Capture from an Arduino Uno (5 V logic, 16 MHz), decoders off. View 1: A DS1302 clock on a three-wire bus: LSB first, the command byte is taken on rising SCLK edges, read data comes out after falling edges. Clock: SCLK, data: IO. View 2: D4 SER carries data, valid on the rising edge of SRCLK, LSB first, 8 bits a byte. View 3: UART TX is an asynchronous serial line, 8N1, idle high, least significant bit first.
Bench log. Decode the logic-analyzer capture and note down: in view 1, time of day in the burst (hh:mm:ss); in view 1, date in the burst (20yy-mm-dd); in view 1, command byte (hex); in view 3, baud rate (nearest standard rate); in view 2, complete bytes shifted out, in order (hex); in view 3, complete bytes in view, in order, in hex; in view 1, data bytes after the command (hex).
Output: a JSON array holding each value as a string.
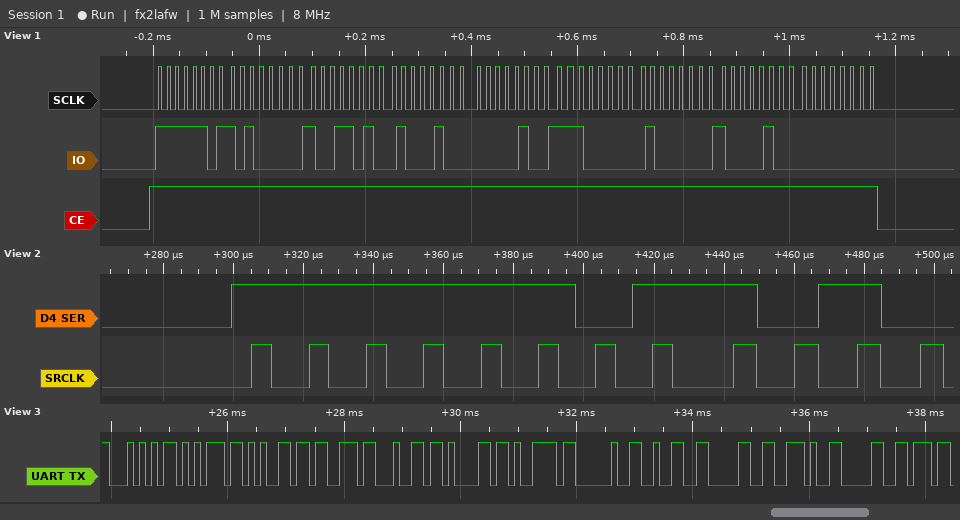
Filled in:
["22:59:05", "2021-07-20", "0xBF", "9600 baud", "BF", "54 75 65 73 64 61 79 20 32 30 2E 30", "05 59 22 20 07 02 21 00"]
